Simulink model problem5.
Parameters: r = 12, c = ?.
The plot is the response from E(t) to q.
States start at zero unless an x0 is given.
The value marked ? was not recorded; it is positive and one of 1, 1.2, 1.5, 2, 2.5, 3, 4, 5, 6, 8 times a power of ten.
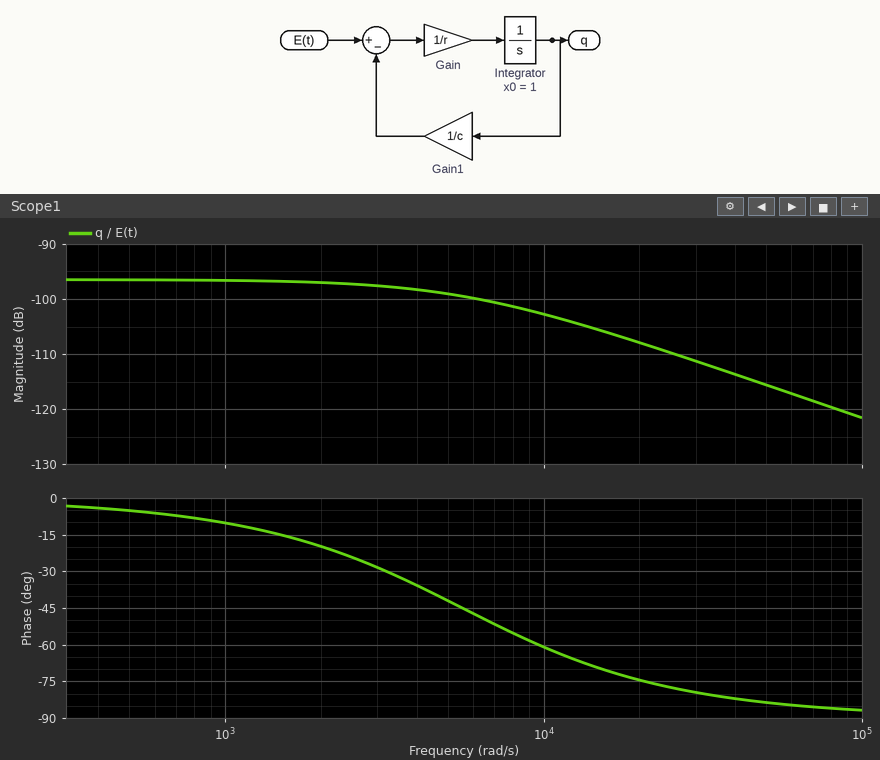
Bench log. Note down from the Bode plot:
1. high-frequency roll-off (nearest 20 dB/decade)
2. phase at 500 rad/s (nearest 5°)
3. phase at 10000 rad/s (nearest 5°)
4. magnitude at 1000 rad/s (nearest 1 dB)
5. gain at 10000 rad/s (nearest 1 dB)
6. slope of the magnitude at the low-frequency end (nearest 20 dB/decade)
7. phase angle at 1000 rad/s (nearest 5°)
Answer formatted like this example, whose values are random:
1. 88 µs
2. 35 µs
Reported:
1. -20 dB/decade
2. -5°
3. -60°
4. -97 dB
5. -103 dB
6. 0 dB/decade
7. -10°
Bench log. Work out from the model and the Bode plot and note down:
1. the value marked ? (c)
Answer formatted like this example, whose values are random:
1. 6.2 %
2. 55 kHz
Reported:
1. 1.5e-05
